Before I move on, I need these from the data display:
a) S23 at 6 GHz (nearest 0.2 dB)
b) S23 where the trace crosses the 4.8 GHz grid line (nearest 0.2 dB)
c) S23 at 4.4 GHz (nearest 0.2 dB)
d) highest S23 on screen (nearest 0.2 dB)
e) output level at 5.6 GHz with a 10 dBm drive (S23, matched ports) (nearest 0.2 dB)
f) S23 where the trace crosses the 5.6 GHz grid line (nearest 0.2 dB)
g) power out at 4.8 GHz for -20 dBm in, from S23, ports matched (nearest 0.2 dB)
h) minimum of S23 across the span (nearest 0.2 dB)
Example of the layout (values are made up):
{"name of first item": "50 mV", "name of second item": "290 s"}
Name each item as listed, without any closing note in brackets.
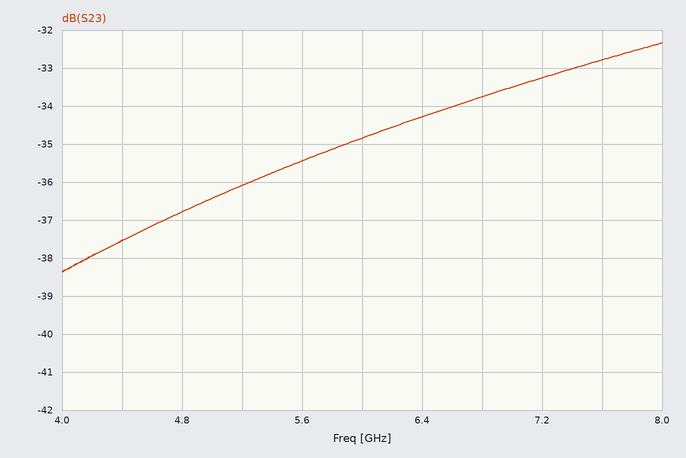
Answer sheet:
{"S23 at 6 GHz": "-34.8 dB", "S23 where the trace crosses the 4.8 GHz grid line": "-36.8 dB", "S23 at 4.4 GHz": "-37.6 dB", "highest S23 on screen": "-32.4 dB", "output level at 5.6 GHz with a 10 dBm drive (S23, matched ports)": "-25.4 dBm", "S23 where the trace crosses the 5.6 GHz grid line": "-35.4 dB", "power out at 4.8 GHz for -20 dBm in, from S23, ports matched": "-56.8 dBm", "minimum of S23 across the span": "-38.4 dB"}
